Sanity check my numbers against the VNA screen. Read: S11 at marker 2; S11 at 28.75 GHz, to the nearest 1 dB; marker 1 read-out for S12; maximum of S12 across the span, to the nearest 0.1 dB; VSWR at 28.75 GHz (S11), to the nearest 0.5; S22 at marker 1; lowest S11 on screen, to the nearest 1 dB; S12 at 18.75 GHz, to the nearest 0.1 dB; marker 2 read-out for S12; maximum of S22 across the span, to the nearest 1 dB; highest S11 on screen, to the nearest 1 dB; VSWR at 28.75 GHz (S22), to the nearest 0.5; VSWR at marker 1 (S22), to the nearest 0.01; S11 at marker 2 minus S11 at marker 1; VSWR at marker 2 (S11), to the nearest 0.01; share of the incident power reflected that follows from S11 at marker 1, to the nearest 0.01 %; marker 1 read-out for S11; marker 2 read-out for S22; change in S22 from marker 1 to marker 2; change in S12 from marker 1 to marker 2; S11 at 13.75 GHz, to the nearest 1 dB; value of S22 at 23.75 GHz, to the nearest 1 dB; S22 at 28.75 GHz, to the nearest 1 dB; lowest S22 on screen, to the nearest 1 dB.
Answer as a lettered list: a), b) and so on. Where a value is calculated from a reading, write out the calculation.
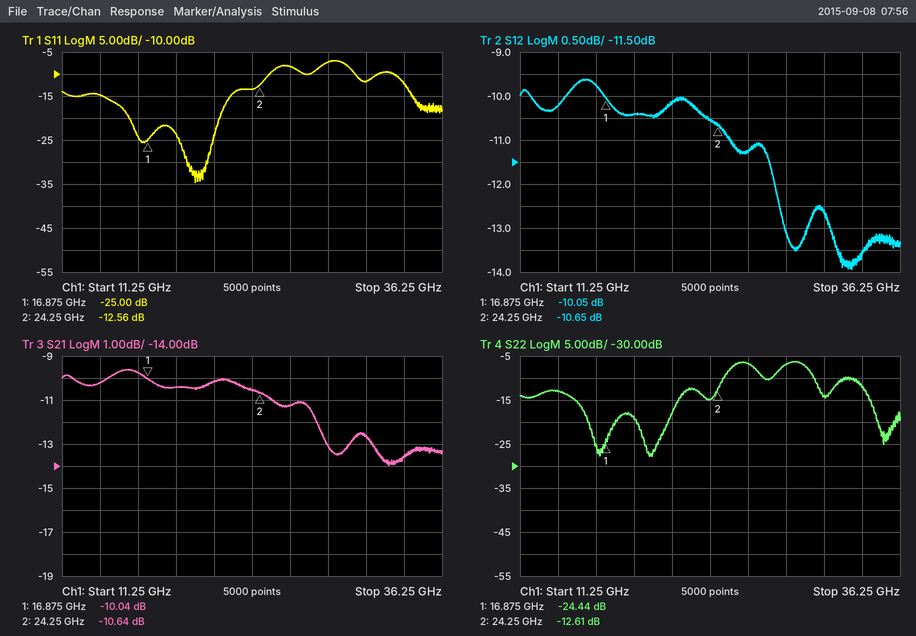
a) -12.56 dB
b) -7 dB
c) -10.05 dB
d) -9.6 dB
e) |Γ| = 10^(-7/20) = 0.4467; VSWR = (1 + 0.4467)/(1 − 0.4467) ≈ 2.61, so 2.5 to the nearest 0.5
f) -24.44 dB
g) -35 dB
h) -10.4 dB
i) -10.65 dB
j) -6 dB
k) -7 dB
l) |Γ| = 10^(-7/20) = 0.4467; VSWR = (1 + 0.4467)/(1 − 0.4467) ≈ 2.61, so 2.5 to the nearest 0.5
m) (1 + 0.0600)/(1 − 0.0600) ≈ 1.13
n) -12.56 − (-25) = 12.44 dB
o) (1 + 0.2355)/(1 − 0.2355) ≈ 1.62
p) 10^(-25/10) ≈ 0.32 %
q) -25.00 dB
r) -12.61 dB
s) -12.61 − (-24.44) = 11.83 dB
t) -10.65 − (-10.05) = -0.60 dB
u) -15 dB
v) -15 dB
w) -7 dB
x) -28 dB
